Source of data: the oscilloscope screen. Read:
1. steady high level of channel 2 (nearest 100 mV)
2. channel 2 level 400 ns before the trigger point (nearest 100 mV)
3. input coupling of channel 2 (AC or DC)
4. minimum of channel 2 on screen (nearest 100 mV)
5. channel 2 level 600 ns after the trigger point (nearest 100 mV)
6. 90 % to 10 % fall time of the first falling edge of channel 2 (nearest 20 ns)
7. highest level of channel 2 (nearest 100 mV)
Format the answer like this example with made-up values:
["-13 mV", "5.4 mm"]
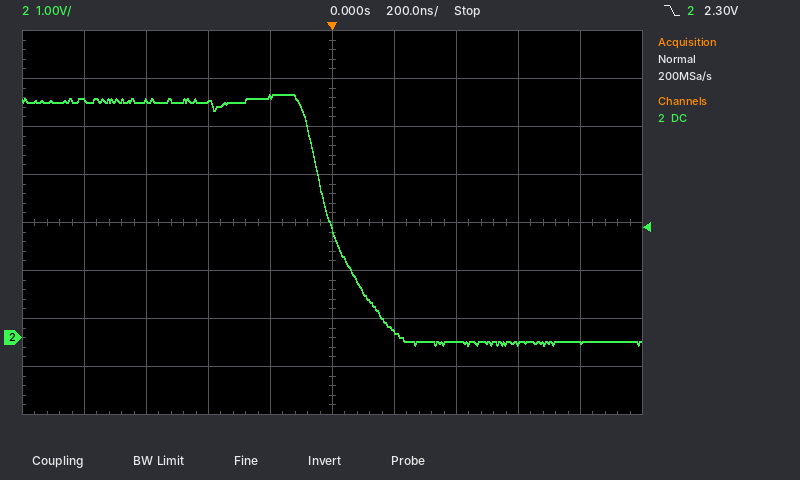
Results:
["4.9 V", "4.9 V", "DC", "-200 mV", "-100 mV", "240 ns", "5.1 V"]
